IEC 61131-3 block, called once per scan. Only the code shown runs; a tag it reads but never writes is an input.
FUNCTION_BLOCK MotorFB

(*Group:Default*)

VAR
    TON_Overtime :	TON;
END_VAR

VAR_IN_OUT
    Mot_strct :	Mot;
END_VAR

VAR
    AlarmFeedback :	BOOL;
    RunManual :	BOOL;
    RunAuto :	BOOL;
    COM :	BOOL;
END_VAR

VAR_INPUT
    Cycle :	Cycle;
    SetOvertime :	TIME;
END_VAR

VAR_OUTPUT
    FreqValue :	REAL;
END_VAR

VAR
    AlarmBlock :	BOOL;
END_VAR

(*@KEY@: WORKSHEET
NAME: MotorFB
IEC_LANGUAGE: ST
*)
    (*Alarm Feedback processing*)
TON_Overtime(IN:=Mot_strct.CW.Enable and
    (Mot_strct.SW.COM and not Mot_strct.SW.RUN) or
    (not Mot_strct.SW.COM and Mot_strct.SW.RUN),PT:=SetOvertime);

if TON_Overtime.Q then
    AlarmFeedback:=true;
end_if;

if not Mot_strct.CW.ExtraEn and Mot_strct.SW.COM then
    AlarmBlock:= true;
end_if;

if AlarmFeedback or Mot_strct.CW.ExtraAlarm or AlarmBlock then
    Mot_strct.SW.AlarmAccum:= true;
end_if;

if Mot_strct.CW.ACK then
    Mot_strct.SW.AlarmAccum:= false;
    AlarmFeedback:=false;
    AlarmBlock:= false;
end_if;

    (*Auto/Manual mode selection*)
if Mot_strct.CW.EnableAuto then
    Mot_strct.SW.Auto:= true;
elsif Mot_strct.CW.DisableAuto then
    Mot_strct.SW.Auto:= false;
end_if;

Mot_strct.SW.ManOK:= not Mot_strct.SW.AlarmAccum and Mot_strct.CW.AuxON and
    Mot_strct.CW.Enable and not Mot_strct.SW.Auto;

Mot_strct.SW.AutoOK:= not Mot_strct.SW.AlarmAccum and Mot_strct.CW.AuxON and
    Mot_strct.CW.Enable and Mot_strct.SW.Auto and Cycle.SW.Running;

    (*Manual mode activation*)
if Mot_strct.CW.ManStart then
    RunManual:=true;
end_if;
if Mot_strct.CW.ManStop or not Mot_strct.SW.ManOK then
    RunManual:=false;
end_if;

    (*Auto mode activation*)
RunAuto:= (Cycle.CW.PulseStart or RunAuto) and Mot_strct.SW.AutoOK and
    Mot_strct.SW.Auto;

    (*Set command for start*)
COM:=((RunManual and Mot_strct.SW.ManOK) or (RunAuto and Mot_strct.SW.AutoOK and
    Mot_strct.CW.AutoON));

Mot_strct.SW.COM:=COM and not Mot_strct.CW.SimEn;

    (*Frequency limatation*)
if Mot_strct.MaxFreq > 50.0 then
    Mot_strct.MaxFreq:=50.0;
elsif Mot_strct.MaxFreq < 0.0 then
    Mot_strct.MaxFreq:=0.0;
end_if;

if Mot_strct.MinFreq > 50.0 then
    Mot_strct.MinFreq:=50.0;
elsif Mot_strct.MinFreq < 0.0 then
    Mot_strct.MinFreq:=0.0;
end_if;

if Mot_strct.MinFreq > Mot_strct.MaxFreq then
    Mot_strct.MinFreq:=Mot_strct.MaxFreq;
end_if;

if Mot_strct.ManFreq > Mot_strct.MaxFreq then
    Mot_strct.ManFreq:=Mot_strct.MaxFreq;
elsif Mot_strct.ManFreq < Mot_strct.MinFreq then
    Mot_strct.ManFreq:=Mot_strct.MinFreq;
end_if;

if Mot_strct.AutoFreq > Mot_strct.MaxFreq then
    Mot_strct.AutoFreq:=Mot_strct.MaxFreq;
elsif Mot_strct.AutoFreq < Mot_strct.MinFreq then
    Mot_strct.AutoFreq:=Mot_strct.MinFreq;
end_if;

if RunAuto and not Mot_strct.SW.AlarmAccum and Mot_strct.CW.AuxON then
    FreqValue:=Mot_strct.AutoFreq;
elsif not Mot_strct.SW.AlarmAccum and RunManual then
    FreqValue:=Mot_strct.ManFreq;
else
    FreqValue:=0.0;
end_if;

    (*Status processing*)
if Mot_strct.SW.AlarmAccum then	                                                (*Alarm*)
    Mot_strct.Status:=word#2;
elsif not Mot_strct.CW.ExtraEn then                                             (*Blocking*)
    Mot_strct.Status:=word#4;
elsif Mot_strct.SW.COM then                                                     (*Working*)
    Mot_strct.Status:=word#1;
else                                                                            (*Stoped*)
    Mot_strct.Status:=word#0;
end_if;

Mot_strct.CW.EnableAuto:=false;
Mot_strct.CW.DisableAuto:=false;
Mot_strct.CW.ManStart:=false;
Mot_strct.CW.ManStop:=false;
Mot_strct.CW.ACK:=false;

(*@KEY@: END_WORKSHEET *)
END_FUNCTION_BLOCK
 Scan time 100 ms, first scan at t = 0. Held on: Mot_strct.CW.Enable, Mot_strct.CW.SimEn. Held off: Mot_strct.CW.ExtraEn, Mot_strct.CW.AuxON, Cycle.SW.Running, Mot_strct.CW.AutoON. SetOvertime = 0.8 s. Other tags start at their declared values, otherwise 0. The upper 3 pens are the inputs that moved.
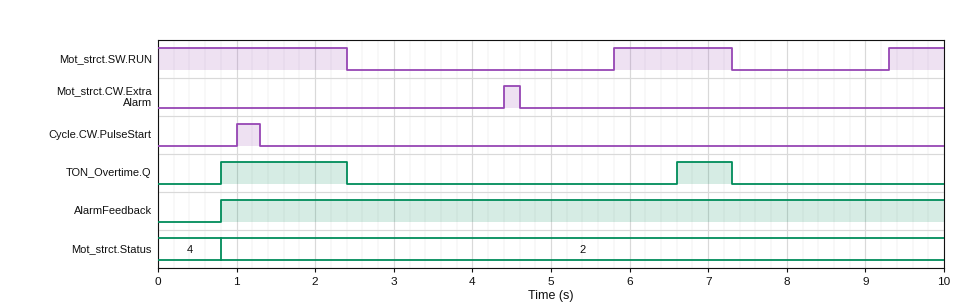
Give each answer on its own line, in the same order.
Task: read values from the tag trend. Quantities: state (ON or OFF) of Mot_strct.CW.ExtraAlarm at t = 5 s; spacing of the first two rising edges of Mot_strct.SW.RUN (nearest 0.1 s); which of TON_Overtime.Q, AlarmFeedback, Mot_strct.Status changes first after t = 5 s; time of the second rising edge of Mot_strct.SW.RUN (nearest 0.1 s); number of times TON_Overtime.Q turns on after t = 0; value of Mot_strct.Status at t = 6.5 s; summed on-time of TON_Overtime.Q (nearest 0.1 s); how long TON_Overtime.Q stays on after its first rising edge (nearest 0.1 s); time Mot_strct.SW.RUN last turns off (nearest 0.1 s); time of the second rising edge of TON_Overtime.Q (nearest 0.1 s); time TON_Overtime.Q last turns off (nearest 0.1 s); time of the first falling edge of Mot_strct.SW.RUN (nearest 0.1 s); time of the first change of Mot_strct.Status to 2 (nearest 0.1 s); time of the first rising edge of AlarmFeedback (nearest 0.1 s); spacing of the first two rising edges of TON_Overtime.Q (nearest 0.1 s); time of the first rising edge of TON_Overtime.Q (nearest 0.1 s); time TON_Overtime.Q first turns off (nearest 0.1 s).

OFF
3.5 s
TON_Overtime.Q
9.3 s
2
2
2.3 s
1.6 s
7.3 s
6.6 s
7.3 s
2.4 s
0.8 s
0.8 s
5.8 s
0.8 s
2.4 s
